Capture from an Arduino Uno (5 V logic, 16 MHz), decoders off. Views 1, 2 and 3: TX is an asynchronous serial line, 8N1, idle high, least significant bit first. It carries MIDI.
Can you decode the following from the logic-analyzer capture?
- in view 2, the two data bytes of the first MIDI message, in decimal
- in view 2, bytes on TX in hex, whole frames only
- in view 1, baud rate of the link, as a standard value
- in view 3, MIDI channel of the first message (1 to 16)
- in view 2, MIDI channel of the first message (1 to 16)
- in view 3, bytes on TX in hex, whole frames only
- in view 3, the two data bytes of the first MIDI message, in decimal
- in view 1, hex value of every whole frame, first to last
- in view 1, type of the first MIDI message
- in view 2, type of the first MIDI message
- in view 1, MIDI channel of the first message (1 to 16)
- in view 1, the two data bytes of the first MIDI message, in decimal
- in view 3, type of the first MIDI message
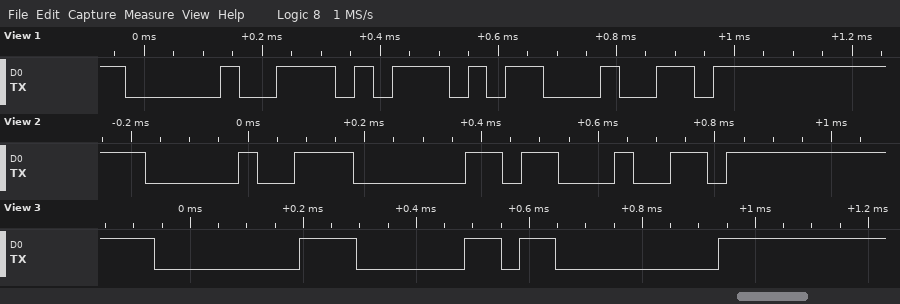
96, 100
90 60 64
31250 baud
1
1
0x80 0x60 0x00
96, 0
0x90 0x5D 0x64
Note On
Note On
1
93, 100
Note Off
